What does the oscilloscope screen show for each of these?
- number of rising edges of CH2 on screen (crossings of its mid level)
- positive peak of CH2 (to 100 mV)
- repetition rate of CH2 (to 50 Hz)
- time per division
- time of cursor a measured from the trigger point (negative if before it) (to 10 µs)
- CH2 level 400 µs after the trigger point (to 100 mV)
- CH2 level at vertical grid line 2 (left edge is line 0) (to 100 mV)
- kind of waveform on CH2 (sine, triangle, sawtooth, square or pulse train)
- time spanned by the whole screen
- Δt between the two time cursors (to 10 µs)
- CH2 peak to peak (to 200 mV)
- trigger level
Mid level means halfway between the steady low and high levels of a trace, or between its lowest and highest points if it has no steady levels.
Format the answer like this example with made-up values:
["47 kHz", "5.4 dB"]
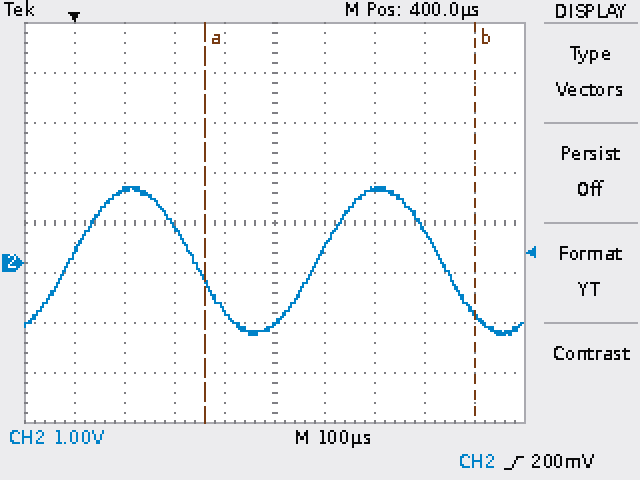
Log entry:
["2", "1.5 V", "2.00 kHz", "100 µs", "+260 µs", "-1.2 V", "1.5 V", "sine", "1 ms", "540 µs", "3.0 V", "200 mV"]
